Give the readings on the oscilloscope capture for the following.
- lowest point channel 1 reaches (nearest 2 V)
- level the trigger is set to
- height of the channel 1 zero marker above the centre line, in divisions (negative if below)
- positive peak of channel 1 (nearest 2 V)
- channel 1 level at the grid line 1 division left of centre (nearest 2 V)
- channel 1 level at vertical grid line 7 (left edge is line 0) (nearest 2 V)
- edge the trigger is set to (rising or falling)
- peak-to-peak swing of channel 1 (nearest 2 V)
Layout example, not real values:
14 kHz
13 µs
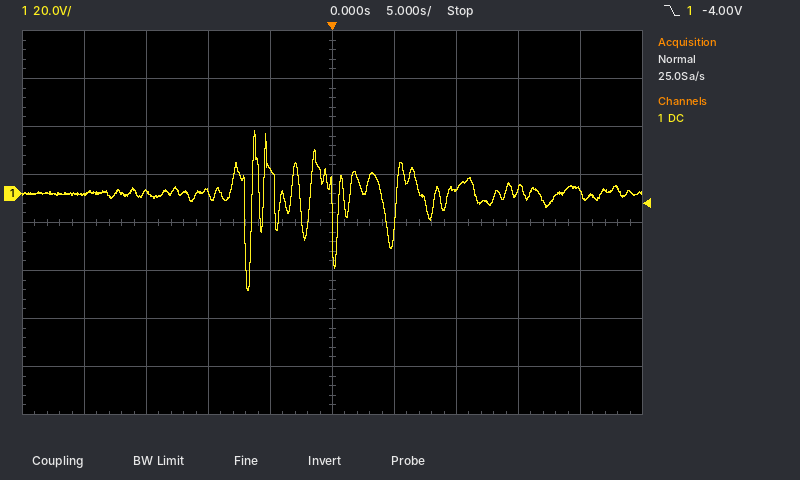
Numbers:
-40 V
-4.00 V
+0.6 div
26 V
10 V
2 V
falling
66 V
